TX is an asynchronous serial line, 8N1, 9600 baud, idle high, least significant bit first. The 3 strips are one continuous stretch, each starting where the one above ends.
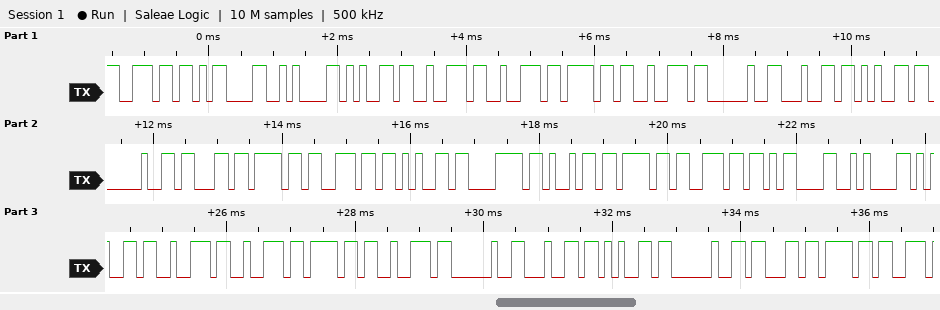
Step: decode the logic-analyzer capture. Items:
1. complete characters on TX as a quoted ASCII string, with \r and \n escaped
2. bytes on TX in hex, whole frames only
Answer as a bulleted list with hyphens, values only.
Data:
- "n\r\nerror de conexion\r\nerror de co"
- 6E 0D 0A 65 72 72 6F 72 20 64 65 20 63 6F 6E 65 78 69 6F 6E 0D 0A 65 72 72 6F 72 20 64 65 20 63 6F
